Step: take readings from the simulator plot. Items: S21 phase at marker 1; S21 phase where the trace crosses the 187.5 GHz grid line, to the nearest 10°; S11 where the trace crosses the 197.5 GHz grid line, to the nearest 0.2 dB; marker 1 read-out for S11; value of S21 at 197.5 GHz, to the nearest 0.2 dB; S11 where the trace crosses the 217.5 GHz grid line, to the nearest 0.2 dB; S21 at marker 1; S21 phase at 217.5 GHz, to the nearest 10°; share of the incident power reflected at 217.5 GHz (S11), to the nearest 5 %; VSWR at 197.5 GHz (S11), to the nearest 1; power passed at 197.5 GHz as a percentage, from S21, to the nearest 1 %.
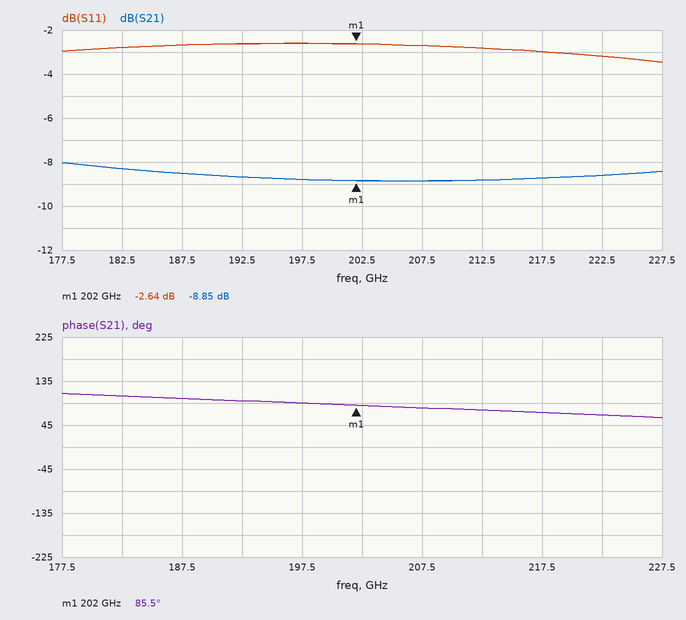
85.5°
100°
-2.6 dB
-2.64 dB
-8.8 dB
-3.0 dB
-8.85 dB
70°
50 %
7
13 %
